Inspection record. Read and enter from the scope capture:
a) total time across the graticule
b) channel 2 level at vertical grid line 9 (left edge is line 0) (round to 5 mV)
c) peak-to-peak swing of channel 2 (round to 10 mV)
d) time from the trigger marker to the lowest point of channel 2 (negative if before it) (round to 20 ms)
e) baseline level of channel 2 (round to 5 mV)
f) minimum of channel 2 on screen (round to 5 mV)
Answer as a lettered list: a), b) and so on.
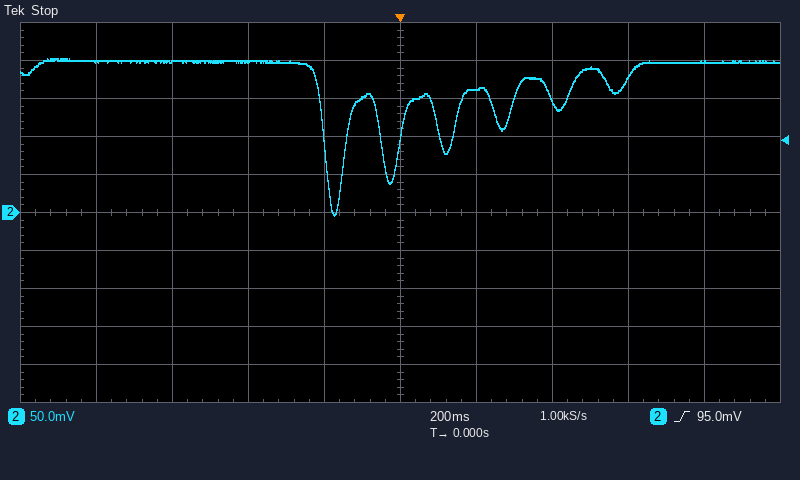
a) 2 s
b) 200 mV
c) 210 mV
d) -180 ms
e) 200 mV
f) -5 mV
